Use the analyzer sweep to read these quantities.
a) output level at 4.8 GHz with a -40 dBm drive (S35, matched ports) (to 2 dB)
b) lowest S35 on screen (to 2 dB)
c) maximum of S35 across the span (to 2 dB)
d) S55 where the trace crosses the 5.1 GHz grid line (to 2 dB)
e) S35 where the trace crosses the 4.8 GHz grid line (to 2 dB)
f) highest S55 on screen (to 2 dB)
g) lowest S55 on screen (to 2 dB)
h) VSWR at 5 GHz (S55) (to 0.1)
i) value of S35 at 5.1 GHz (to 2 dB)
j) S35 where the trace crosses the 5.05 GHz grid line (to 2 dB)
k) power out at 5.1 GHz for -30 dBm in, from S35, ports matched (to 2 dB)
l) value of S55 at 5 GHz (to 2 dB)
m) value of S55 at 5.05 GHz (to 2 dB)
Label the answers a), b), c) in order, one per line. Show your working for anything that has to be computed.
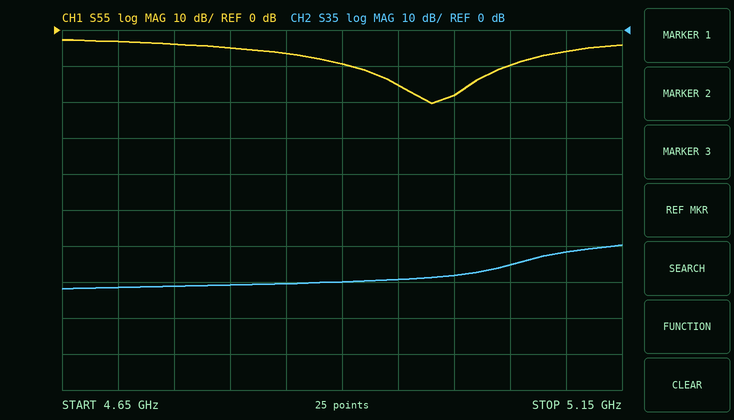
a) -40 dBm + (-70 dB) = -110 dBm
b) -72 dB
c) -60 dB
d) -6 dB
e) -70 dB
f) -2 dB
g) -20 dB
h) |Γ| = 10^(-18/20) = 0.1259; VSWR = (1 + 0.1259)/(1 − 0.1259) ≈ 1.3
i) -62 dB
j) -66 dB
k) -30 dBm + (-62 dB) = -92 dBm
l) -18 dB
m) -10 dB
